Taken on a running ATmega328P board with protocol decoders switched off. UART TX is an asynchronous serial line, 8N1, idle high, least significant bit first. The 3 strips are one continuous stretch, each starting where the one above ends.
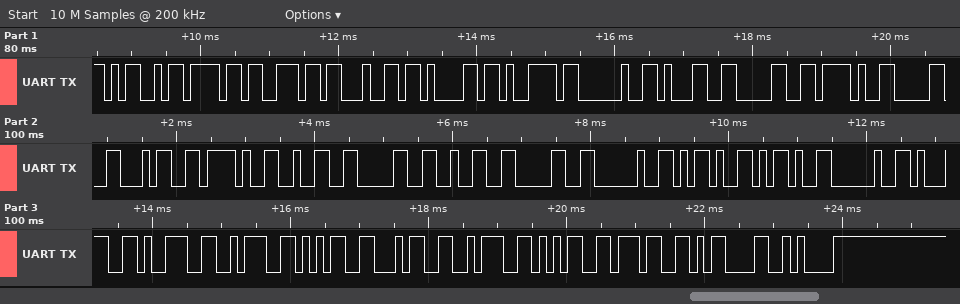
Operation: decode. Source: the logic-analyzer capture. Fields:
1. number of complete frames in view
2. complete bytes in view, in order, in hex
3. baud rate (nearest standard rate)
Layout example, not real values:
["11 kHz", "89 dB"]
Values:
["31", "4D 6F 6E 64 61 79 20 31 30 2F 30 34 2F 32 30 32 30 20 2D 2D 20 31 39 3A 35 34 3A 35 37 0D 0A", "9600 baud"]
